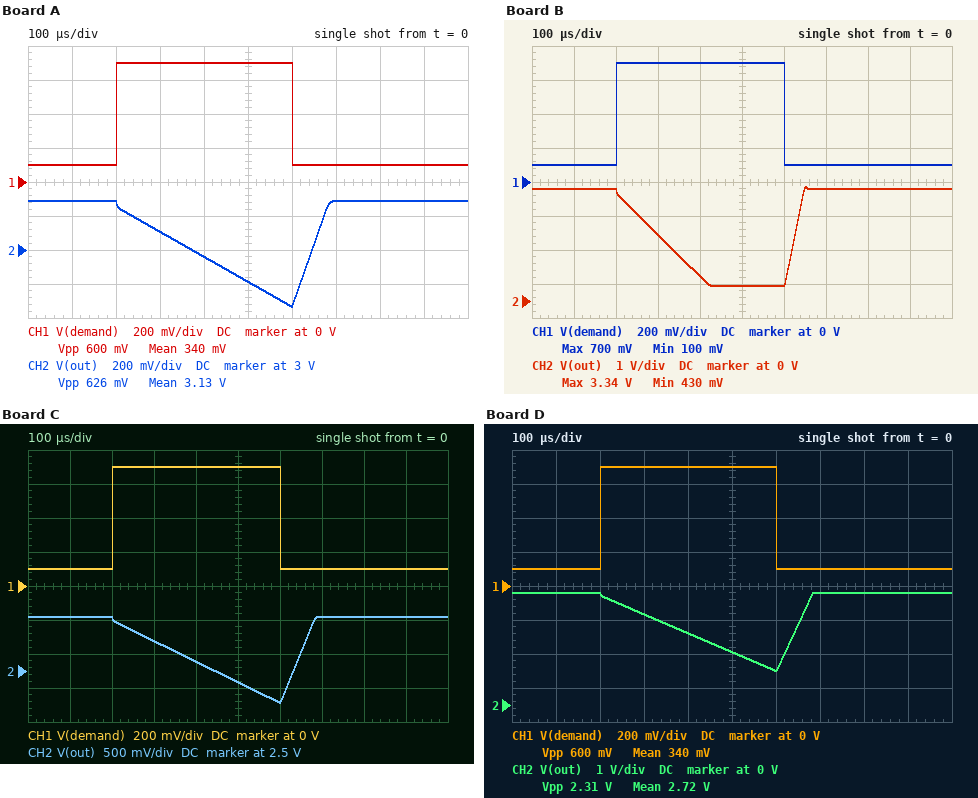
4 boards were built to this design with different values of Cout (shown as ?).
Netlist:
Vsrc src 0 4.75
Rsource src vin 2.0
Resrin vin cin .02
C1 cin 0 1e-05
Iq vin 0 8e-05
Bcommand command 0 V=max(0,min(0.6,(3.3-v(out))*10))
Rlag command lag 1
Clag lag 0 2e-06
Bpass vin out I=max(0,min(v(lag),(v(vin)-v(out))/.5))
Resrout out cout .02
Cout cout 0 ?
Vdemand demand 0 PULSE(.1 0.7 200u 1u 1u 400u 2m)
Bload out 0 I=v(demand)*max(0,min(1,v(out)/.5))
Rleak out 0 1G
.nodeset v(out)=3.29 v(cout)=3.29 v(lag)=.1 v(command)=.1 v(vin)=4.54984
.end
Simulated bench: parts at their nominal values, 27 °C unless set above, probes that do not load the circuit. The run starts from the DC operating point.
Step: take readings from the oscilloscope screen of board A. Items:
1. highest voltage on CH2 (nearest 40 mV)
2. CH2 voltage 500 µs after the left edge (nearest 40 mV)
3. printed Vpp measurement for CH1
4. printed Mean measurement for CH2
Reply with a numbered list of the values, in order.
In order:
1. 3.28 V
2. 2.80 V
3. 600 mV
4. 3.13 V
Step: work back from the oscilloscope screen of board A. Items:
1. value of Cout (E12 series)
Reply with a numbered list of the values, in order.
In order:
1. 68 µF
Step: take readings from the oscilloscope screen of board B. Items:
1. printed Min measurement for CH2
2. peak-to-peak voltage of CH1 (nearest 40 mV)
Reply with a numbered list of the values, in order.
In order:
1. 430 mV
2. 600 mV
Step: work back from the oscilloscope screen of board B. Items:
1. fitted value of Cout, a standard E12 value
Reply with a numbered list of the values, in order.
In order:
1. 8.2 µF
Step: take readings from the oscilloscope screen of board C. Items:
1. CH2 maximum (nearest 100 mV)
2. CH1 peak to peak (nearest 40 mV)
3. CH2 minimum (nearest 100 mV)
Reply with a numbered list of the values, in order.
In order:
1. 3.3 V
2. 600 mV
3. 2.0 V
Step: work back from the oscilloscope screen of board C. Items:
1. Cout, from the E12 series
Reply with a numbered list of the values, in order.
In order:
1. 33 µF
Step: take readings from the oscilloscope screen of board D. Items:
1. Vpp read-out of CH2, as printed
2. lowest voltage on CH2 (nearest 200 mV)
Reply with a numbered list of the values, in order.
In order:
1. 2.31 V
2. 1.0 V
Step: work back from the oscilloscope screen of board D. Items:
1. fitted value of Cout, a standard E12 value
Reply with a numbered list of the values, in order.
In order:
1. 18 µF
